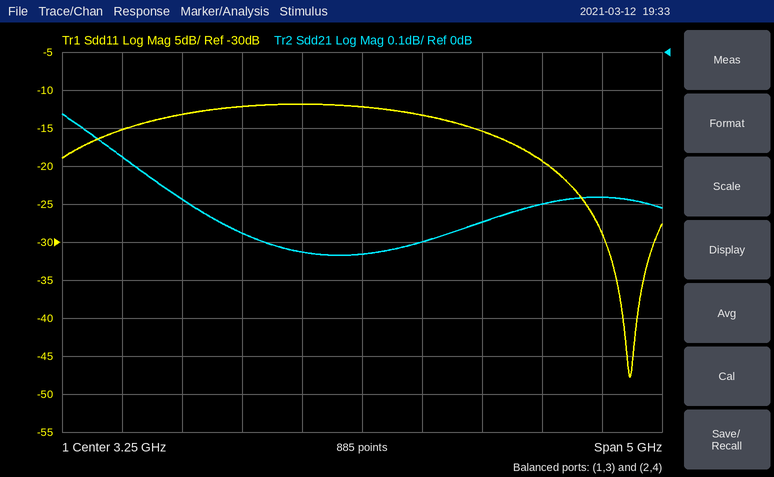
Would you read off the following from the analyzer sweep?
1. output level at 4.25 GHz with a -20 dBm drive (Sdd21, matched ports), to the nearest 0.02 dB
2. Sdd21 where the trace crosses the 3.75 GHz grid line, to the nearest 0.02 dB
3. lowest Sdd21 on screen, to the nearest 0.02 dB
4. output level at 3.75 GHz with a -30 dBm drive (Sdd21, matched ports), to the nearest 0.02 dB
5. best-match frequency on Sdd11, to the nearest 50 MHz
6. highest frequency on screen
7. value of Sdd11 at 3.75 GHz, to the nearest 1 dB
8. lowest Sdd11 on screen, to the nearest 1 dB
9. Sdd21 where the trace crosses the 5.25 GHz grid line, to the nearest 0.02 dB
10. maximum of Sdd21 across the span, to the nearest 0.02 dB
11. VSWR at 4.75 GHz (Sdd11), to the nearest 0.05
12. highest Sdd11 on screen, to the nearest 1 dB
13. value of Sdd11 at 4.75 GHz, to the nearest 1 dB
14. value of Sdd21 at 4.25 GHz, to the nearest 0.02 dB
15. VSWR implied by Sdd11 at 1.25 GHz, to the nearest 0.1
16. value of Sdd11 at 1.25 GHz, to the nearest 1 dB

-20.44 dBm
-0.50 dB
-0.54 dB
-30.50 dBm
5.50 GHz
5.75 GHz
-13 dB
-48 dB
-0.38 dB
-0.16 dB
1.25
-12 dB
-19 dB
-0.44 dB
1.4
-15 dB
